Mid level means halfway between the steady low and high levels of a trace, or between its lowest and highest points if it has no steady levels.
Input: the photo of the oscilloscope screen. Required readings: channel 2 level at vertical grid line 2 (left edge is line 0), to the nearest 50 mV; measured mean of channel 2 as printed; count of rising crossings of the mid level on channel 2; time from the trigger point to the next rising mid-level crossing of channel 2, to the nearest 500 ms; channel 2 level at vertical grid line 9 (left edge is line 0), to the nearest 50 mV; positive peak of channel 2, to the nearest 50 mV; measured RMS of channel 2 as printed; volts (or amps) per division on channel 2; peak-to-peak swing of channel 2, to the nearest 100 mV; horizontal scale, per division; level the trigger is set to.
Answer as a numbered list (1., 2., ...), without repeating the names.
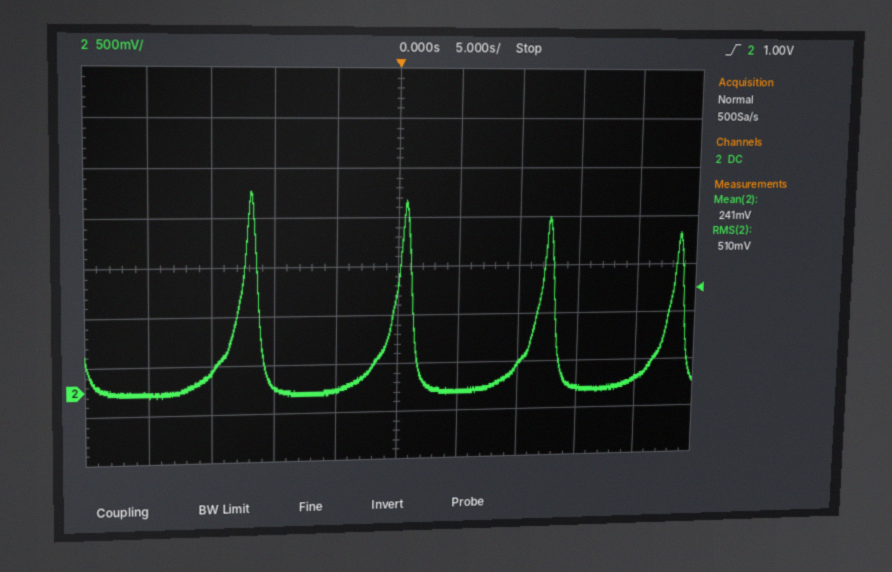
1. 200 mV
2. 241 mV
3. 4
4. 12.0 s
5. 50 mV
6. 2.00 V
7. 510 mV
8. 500 mV
9. 2.10 V
10. 5 s
11. 1.00 V
